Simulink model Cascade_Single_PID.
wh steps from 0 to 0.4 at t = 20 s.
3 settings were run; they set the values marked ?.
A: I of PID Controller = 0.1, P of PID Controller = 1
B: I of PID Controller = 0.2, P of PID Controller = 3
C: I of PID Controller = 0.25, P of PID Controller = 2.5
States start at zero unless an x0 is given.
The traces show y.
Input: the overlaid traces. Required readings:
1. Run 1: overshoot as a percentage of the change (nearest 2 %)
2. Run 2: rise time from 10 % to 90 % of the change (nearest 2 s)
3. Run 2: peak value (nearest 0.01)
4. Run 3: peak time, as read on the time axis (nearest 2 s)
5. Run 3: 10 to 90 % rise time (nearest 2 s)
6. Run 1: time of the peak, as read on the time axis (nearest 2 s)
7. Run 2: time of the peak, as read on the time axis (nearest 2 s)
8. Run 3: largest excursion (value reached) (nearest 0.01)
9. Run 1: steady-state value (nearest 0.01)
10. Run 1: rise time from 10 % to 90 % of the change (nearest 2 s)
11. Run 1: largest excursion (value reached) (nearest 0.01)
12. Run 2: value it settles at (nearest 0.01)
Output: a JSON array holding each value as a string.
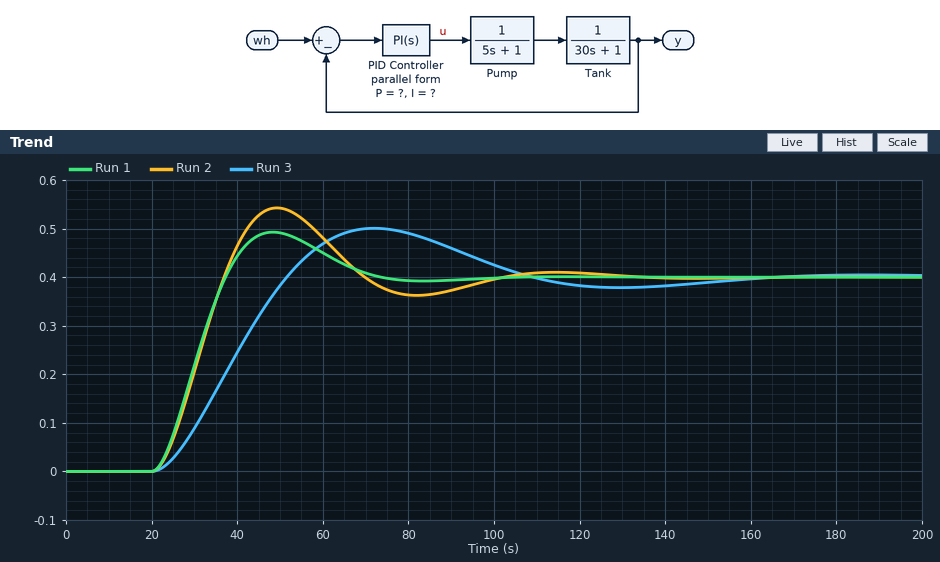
["24 %", "12 s", "0.54", "72 s", "22 s", "48 s", "50 s", "0.50", "0.40", "12 s", "0.49", "0.40"]
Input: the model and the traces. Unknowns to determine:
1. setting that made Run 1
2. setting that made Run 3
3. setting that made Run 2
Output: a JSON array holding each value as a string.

["B", "A", "C"]
